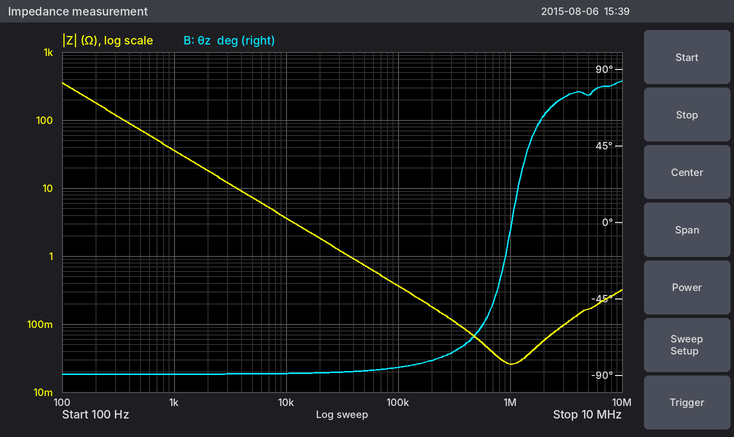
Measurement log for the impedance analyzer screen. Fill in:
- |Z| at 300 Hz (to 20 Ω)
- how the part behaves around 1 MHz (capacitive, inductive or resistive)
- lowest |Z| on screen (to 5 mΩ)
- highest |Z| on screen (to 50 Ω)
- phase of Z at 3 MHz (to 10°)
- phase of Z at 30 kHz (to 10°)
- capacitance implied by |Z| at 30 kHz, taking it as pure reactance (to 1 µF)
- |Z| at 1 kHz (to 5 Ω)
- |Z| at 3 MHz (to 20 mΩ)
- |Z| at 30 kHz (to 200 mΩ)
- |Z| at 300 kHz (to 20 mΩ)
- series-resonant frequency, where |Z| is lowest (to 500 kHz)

120 Ω
resistive
25 mΩ
350 Ω
70°
-90°
4 µF
35 Ω
100 mΩ
1.2 Ω
120 mΩ
1.0 MHz
